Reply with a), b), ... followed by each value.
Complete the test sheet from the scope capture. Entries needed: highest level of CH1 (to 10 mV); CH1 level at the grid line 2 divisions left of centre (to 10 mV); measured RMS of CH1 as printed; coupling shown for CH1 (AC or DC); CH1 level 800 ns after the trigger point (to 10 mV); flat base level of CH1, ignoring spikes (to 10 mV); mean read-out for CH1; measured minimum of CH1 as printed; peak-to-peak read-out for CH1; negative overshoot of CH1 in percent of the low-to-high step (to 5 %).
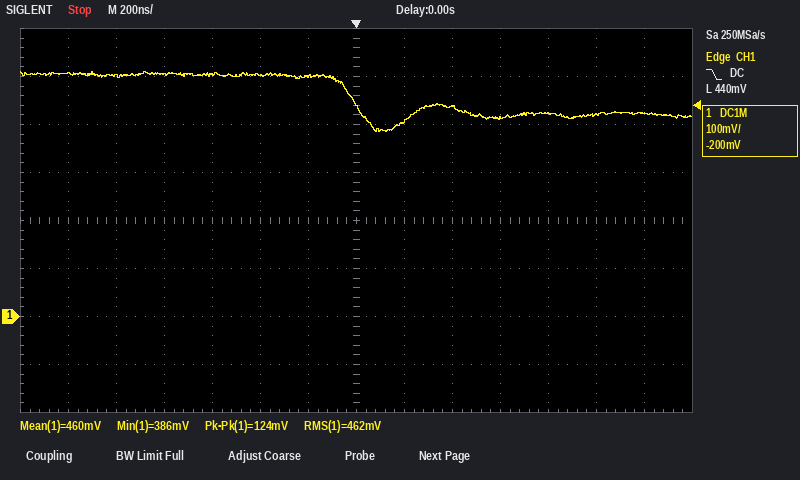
a) 510 mV
b) 500 mV
c) 462 mV
d) DC
e) 420 mV
f) 420 mV
g) 460 mV
h) 386 mV
i) 124 mV
j) 40 %
